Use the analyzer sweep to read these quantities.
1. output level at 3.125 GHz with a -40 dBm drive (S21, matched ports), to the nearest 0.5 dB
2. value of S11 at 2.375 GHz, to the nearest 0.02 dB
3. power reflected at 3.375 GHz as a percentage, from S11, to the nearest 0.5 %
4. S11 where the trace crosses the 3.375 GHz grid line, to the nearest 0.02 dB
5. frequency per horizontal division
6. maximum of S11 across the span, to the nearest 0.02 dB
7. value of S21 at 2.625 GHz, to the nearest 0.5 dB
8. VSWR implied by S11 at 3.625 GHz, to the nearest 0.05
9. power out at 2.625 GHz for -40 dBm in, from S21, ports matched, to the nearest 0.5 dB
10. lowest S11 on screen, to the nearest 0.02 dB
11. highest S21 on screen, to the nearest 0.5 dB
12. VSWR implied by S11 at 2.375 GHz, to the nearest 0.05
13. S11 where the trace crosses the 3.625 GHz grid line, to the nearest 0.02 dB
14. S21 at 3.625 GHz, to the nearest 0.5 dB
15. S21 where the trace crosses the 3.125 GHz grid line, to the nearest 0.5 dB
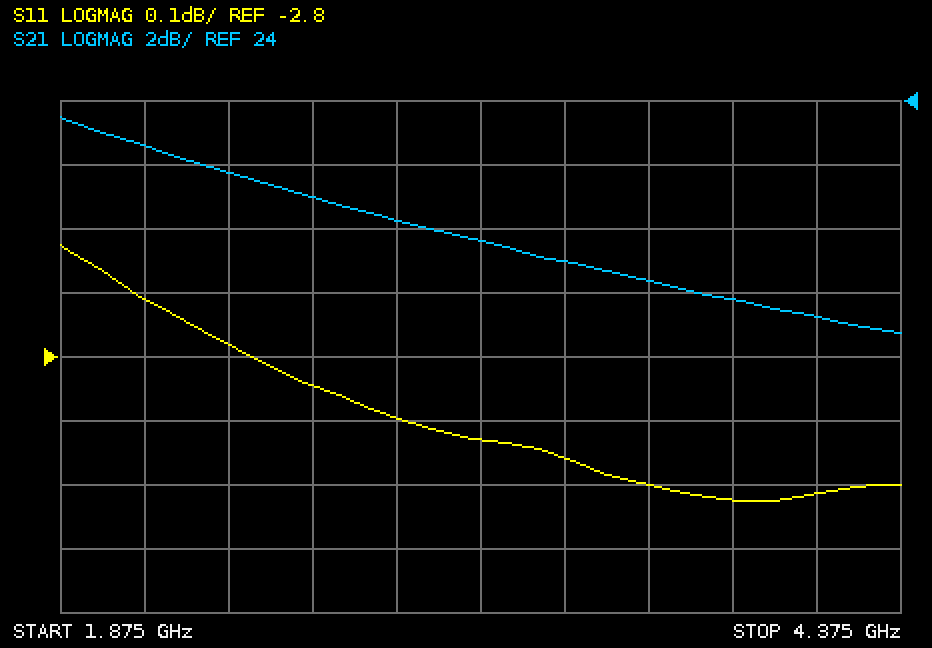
-20.5 dBm
-2.78 dB
50.5 %
-2.96 dB
250 MHz
-2.62 dB
21.0 dB
5.85
-19.0 dBm
-3.02 dB
23.5 dB
6.30
-3.00 dB
18.5 dB
19.5 dB
